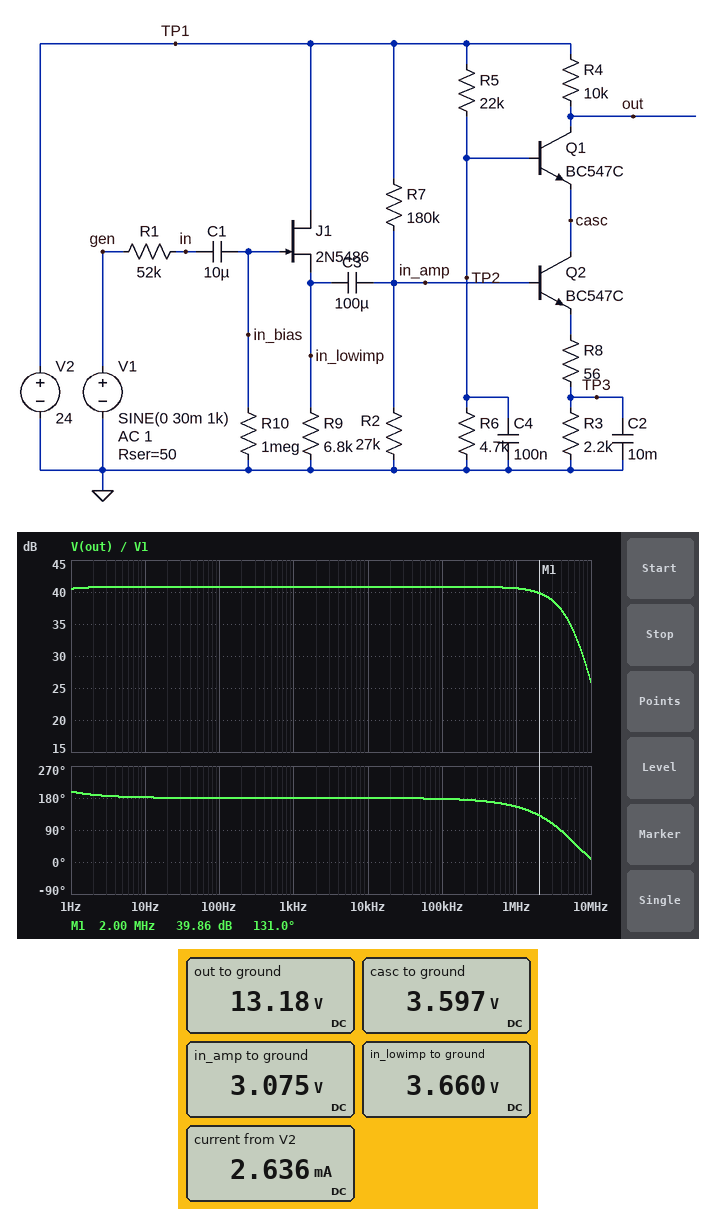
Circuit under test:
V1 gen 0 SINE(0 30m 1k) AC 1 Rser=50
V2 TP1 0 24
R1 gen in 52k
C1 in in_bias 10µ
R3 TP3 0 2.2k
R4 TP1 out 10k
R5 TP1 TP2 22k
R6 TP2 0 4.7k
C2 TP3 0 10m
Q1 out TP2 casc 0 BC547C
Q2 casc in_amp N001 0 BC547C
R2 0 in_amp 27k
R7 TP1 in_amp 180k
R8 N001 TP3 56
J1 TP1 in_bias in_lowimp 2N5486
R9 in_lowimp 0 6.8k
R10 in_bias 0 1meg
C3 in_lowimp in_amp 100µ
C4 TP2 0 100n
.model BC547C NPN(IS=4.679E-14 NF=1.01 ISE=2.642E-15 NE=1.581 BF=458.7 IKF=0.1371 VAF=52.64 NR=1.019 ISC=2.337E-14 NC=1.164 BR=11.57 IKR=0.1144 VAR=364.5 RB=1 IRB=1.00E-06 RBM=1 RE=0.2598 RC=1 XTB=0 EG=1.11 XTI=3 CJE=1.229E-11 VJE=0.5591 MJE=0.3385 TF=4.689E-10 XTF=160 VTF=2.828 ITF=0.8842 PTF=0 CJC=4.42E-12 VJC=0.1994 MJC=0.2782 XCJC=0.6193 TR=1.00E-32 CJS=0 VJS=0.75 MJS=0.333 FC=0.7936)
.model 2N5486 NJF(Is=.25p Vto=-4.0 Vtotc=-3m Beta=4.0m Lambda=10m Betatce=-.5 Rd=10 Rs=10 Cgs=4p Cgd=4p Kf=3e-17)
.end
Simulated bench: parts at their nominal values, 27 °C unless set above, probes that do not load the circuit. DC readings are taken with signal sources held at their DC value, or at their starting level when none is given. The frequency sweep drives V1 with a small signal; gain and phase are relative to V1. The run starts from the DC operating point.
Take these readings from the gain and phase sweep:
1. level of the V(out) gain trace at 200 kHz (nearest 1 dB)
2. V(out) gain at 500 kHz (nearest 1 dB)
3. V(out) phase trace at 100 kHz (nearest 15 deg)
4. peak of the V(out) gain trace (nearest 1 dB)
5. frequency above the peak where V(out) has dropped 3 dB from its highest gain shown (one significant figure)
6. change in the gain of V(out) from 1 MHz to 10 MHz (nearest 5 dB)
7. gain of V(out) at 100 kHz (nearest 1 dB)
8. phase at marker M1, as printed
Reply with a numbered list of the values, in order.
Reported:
1. 41 dB
2. 41 dB
3. 180 deg
4. 41 dB
5. 4 MHz
6. -15 dB
7. 41 dB
8. 131.0 deg
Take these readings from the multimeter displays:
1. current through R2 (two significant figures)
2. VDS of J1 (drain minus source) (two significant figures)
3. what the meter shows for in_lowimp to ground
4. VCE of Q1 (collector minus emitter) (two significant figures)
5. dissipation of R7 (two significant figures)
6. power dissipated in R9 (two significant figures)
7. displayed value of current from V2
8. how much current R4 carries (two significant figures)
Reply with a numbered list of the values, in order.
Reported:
1. 110 µA
2. 20 V
3. 3.660 V
4. 9.6 V
5. 2.4 mW
6. 2.0 mW
7. 2.636 mA
8. 1.1 mA
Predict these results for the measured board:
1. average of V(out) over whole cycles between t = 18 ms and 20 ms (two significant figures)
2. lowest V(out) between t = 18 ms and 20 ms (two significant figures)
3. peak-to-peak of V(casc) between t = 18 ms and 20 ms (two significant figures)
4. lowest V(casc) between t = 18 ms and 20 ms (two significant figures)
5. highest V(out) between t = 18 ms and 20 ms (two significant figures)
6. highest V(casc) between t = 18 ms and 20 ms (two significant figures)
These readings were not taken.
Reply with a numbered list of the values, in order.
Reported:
1. 13 V
2. 9.8 V
3. 20 mV
4. 3.6 V
5. 16 V
6. 3.6 V
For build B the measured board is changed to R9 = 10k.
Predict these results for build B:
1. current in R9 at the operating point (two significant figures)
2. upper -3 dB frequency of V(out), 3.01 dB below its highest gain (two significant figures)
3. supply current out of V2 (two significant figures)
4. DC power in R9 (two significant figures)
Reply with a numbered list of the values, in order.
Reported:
1. 370 µA
2. 3.7 MHz
3. 2.5 mA
4. 1.4 mW
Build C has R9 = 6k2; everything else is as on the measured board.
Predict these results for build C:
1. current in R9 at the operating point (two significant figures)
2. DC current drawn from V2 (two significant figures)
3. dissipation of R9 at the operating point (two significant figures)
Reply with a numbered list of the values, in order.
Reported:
1. 590 µA
2. 2.7 mA
3. 2.1 mW
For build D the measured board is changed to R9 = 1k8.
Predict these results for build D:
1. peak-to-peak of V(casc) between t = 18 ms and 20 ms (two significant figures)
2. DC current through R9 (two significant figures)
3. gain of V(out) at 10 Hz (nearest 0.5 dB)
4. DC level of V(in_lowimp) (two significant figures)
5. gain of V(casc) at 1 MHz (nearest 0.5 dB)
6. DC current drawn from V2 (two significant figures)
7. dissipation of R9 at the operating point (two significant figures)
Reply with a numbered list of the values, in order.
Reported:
1. 19 mV
2. 1.9 mA
3. 40.5 dB
4. 3.4 V
5. -10.5 dB
6. 4.0 mA
7. 6.3 mW
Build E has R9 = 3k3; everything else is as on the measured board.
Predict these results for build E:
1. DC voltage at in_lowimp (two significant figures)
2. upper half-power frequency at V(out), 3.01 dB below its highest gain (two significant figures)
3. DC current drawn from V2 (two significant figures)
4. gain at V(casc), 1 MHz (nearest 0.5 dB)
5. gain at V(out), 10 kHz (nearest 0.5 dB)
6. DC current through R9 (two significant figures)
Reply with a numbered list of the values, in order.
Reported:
1. 3.5 V
2. 3.4 MHz
3. 3.2 mA
4. -10.5 dB
5. 40.5 dB
6. 1.1 mA
